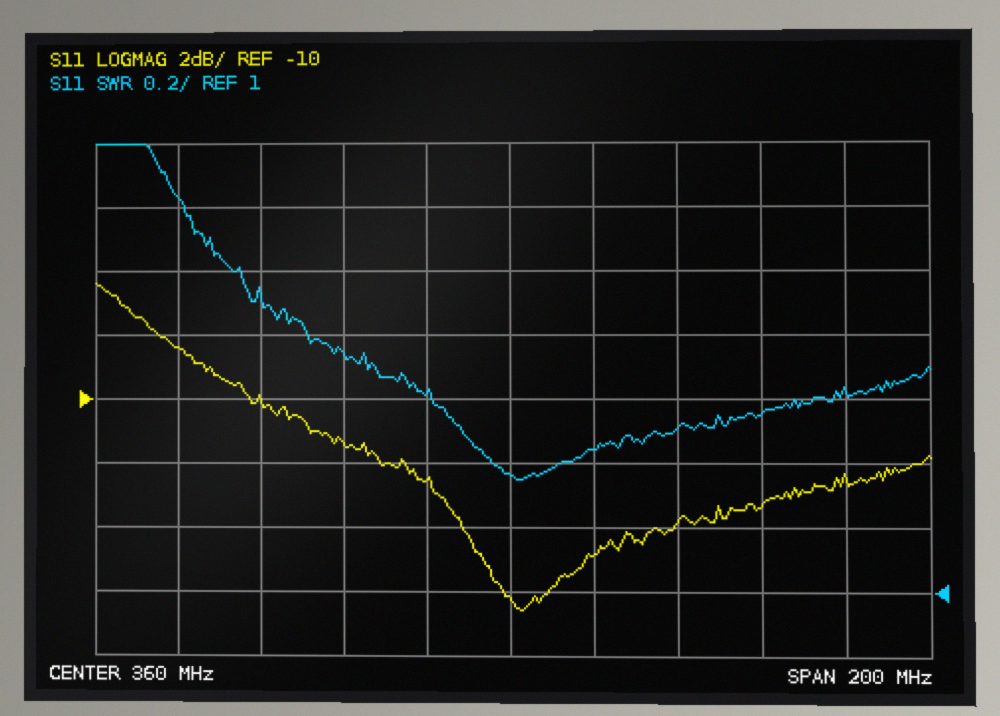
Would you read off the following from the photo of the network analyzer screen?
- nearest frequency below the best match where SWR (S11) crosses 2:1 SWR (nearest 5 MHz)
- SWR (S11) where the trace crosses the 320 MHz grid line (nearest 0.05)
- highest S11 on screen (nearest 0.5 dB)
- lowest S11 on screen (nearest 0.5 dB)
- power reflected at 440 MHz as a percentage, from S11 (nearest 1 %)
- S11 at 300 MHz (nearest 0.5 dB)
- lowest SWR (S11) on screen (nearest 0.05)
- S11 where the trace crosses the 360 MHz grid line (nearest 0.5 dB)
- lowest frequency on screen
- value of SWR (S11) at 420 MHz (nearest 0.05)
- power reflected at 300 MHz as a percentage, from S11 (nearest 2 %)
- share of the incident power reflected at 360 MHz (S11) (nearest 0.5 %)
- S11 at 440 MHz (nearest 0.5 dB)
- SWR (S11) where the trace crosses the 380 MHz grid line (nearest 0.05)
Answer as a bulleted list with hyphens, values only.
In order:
- 295 MHz
- 1.75
- -6.5 dB
- -16.5 dB
- 6 %
- -10.0 dB
- 1.35
- -16.0 dB
- 260 MHz
- 1.55
- 10 %
- 2.5 %
- -12.5 dB
- 1.45
